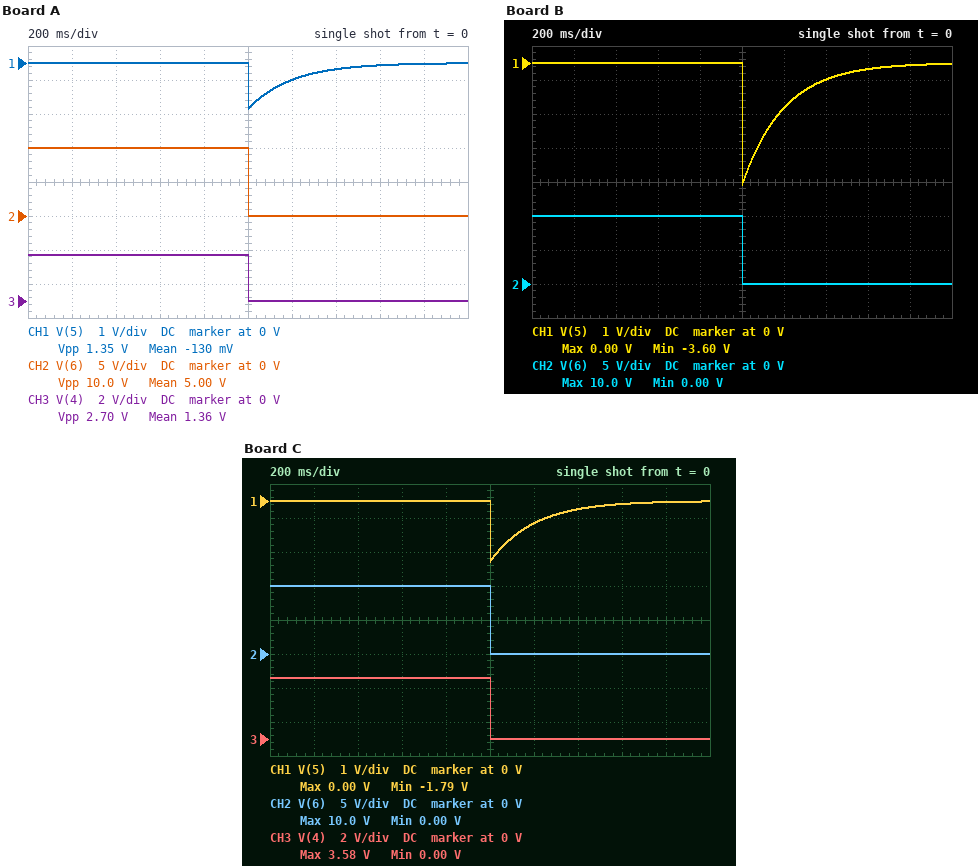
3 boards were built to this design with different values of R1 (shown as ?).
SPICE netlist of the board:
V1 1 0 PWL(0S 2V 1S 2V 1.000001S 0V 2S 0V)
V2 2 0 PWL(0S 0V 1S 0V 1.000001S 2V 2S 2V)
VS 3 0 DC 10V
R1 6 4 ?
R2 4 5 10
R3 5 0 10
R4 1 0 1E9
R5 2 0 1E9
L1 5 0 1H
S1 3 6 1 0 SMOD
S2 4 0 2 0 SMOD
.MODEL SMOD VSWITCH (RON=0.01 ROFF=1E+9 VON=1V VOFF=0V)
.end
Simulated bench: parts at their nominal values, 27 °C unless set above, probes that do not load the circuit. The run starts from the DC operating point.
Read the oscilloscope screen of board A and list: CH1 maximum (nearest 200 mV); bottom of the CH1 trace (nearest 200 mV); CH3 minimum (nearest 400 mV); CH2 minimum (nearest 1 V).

0 V
-1.4 V
0 V
0 V
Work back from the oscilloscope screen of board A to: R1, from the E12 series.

27 Ω
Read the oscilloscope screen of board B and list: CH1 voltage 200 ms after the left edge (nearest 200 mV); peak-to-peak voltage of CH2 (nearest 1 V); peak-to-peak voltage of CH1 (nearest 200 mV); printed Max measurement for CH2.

0 V
10 V
3.6 V
10.0 V
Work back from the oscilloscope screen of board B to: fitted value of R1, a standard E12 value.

3.9 Ω
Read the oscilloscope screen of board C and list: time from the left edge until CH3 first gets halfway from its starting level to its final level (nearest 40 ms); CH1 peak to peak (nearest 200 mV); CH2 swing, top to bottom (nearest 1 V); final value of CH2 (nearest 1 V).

1.00 s
1.8 V
10 V
0 V
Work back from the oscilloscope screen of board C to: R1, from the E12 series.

18 Ω
